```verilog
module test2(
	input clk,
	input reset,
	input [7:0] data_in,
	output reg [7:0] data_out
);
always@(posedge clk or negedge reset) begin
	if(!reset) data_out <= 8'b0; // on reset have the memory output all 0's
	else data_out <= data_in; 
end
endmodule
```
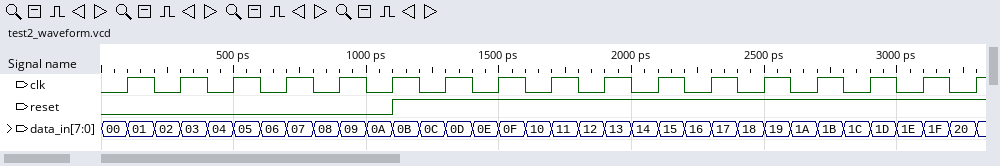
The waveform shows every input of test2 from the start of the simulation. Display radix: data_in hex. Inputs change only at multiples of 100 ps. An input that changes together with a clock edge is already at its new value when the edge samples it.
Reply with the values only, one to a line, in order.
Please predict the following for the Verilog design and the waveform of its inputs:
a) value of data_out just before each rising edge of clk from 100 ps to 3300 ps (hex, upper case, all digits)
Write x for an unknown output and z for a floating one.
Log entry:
00, 00, 00, 00, 00, 00, 0B, 0D, 0F, 11, 13, 15, 17, 19, 1B, 1D, 1F
